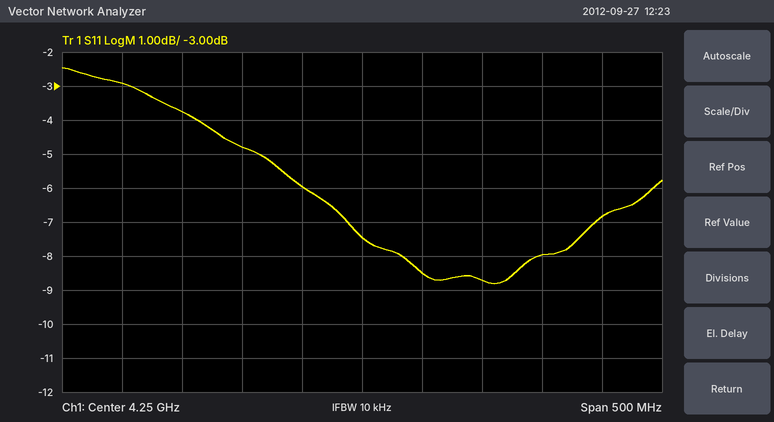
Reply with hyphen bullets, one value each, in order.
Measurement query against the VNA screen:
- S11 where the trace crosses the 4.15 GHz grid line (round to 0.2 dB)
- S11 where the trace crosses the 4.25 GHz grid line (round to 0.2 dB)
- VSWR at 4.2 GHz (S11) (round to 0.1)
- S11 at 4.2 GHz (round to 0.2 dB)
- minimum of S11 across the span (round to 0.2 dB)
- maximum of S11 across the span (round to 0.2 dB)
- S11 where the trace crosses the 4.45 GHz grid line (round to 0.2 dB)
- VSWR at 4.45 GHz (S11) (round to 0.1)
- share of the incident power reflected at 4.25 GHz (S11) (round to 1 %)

- -4.8 dB
- -7.4 dB
- 3.0
- -6.0 dB
- -8.8 dB
- -2.4 dB
- -6.8 dB
- 2.7
- 18 %
